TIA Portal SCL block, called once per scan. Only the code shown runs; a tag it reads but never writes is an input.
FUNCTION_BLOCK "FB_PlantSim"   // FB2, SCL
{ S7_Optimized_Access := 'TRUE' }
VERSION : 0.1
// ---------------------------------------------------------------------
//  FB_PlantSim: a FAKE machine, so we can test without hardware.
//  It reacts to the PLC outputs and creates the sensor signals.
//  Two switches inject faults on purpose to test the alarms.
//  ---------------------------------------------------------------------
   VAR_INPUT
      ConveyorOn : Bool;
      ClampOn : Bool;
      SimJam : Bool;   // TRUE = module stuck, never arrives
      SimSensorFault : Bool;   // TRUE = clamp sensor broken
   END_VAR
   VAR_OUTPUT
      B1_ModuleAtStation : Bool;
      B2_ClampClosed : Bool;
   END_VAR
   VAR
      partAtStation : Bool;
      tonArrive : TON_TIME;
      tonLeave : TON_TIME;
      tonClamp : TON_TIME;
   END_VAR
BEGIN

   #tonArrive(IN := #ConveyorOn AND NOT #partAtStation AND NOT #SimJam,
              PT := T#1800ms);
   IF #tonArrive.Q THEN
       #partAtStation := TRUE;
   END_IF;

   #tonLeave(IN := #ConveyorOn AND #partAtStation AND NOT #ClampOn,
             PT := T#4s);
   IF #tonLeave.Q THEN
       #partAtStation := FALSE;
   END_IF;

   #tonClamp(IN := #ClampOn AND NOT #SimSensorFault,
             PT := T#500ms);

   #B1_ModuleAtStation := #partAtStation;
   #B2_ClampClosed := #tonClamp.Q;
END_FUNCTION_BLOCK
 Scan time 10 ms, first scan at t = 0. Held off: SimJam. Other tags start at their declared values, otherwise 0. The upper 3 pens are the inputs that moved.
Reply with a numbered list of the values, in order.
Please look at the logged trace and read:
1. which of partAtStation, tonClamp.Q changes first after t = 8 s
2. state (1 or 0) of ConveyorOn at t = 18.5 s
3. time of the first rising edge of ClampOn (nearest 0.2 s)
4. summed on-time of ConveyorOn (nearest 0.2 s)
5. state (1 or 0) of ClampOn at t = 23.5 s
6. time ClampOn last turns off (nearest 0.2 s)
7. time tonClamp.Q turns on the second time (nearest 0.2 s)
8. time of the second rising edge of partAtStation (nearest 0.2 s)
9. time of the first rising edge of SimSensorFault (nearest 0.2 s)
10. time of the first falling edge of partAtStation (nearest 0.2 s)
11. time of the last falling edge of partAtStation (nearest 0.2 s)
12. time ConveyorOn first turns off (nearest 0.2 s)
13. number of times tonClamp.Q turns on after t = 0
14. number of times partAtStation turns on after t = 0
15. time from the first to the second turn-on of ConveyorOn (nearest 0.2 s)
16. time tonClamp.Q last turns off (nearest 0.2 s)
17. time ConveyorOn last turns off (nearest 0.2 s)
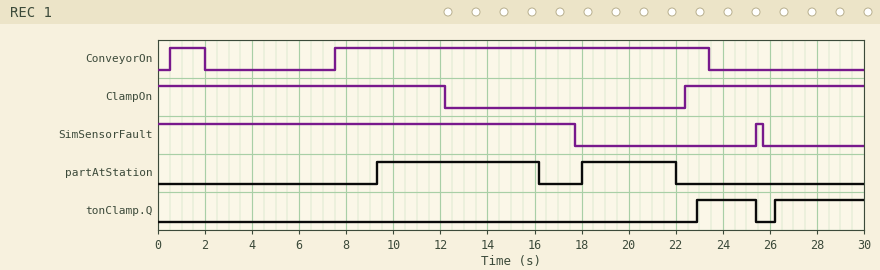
1. partAtStation
2. 1
3. 22.4 s
4. 17.4 s
5. 1
6. 12.2 s
7. 26.2 s
8. 18.0 s
9. 25.4 s
10. 16.2 s
11. 22.0 s
12. 2.0 s
13. 2
14. 2
15. 7.0 s
16. 25.4 s
17. 23.4 s
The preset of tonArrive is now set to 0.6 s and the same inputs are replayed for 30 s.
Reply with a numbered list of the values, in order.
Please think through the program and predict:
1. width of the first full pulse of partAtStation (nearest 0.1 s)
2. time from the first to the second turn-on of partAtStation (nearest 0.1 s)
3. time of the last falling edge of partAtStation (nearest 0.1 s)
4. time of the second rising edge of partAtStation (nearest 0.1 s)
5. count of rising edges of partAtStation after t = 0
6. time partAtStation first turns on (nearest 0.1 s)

1. 15.1 s
2. 15.7 s
3. 20.8 s
4. 16.8 s
5. 3
6. 1.1 s
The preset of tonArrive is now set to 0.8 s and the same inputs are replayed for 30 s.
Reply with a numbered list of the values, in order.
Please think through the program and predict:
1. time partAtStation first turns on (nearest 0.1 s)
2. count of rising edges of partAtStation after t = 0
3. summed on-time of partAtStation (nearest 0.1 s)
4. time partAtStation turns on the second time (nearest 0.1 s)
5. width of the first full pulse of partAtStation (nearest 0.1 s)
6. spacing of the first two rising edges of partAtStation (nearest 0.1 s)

1. 1.3 s
2. 3
3. 27.1 s
4. 17.0 s
5. 14.9 s
6. 15.7 s
